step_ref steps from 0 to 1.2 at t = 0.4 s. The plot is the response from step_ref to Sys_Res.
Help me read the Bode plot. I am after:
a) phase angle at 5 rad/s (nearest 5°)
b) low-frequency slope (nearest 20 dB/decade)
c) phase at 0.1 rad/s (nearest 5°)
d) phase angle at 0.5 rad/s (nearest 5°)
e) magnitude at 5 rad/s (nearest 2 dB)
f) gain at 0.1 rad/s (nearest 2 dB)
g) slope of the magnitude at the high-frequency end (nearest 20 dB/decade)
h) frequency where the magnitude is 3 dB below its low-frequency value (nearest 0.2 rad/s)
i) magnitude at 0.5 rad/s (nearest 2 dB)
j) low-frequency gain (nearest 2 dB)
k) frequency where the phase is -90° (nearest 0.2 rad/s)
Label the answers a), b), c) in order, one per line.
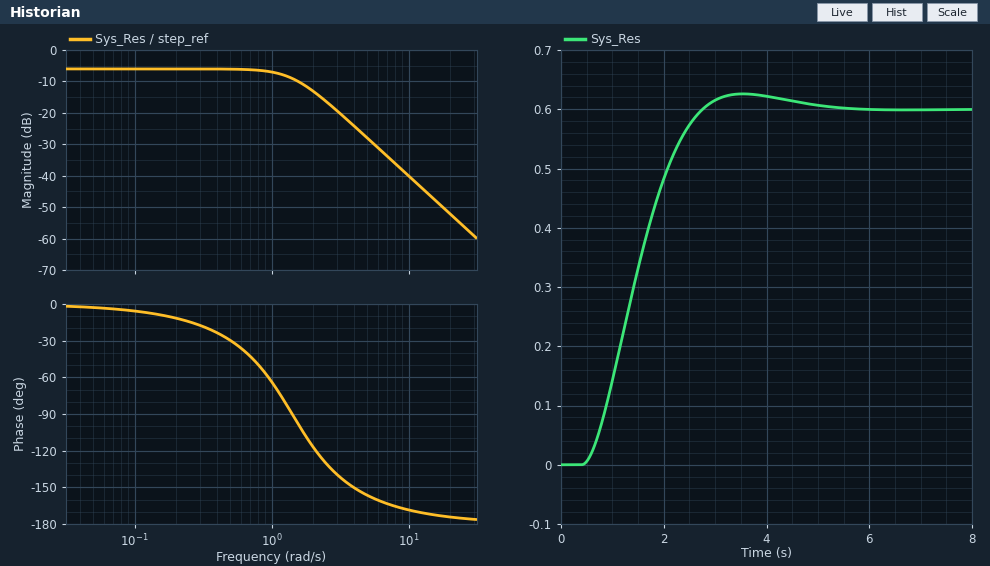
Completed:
a) -155°
b) 0 dB/decade
c) -5°
d) -30°
e) -28 dB
f) -6 dB
g) -40 dB/decade
h) 1.4 rad/s
i) -6 dB
j) -6 dB
k) 1.4 rad/s
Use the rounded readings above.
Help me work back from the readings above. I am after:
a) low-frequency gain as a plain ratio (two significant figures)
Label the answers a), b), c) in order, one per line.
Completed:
a) 0.50
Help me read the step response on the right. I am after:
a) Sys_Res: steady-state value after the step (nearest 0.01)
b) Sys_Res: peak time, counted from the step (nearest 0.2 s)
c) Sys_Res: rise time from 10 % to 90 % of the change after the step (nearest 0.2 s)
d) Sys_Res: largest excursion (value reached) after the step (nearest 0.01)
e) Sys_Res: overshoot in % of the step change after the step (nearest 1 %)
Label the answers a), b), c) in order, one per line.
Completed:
a) 0.60
b) 3.2 s
c) 1.6 s
d) 0.63
e) 4 %
